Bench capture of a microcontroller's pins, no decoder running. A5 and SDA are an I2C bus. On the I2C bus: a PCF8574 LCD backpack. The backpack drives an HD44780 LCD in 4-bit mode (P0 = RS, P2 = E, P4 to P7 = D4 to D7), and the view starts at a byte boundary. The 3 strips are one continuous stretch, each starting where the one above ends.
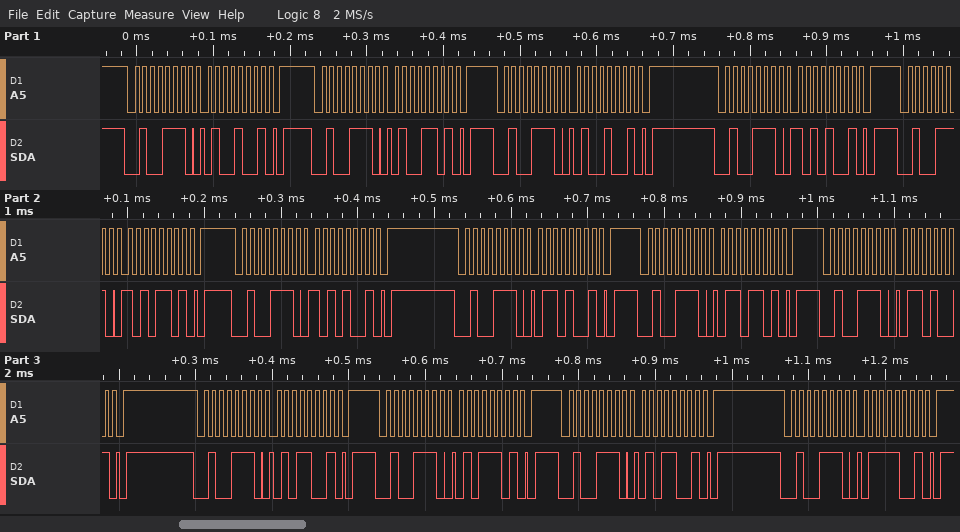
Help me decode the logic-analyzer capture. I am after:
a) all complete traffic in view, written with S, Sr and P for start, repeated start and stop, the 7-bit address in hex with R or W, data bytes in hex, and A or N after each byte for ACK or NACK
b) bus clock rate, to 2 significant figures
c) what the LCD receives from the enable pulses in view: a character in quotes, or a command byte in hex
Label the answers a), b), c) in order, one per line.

a) S 27W A 49 A P S 27W A 4D A P S 27W A 49 A P S 27W A A9 A P S 27W A AD A P S 27W A A9 A P S 27W A 69 A P S 27W A 6D A P S 27W A 69 A P S 27W A 59 A P S 27W A 5D A P S 27W A 59 A P S 27W A 79 A P
b) 100 kHz
c) 'J' 'e'
